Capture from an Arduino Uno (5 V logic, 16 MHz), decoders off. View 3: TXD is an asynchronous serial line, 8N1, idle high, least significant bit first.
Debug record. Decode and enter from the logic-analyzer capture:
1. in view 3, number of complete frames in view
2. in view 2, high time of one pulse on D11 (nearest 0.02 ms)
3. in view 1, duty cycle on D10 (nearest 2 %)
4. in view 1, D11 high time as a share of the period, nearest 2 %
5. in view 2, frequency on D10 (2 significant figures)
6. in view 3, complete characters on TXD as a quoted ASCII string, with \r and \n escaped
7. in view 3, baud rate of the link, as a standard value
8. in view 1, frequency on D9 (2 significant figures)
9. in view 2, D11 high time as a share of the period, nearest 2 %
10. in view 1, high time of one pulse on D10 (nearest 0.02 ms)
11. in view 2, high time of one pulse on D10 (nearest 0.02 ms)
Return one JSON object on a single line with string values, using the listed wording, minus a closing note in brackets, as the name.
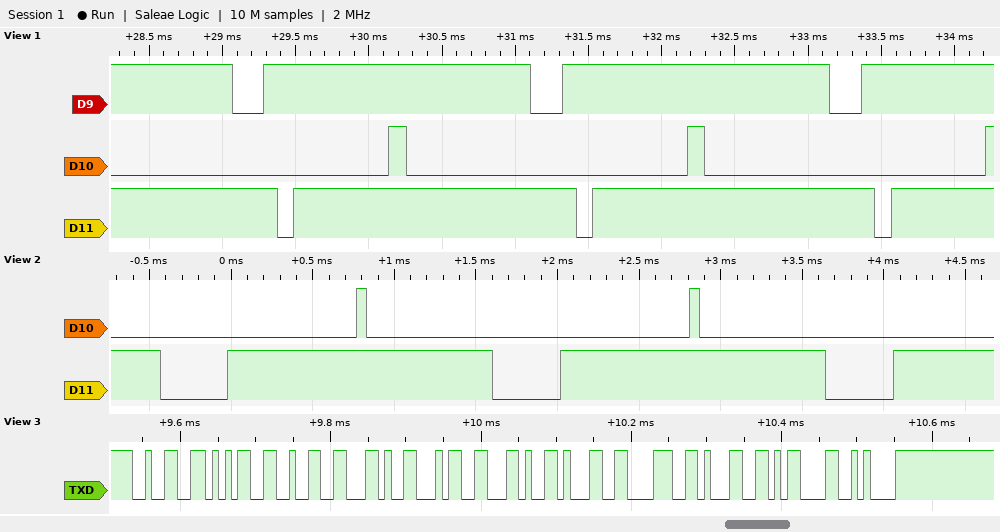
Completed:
{"in view 3, number of complete frames in view": "11", "in view 2, high time of one pulse on D11": "1.62 ms", "in view 1, duty cycle on D10": "6 %", "in view 1, D11 high time as a share of the period, nearest 2 %": "94 %", "in view 2, frequency on D10": "490 Hz", "in view 3, complete characters on TXD as a quoted ASCII string, with \\r and \\n escaped": "\"252,4,181\\r\\n\"", "in view 3, baud rate of the link, as a standard value": "115200 baud", "in view 1, frequency on D9": "490 Hz", "in view 2, D11 high time as a share of the period, nearest 2 %": "80 %", "in view 1, high time of one pulse on D10": "0.12 ms", "in view 2, high time of one pulse on D10": "0.06 ms"}
